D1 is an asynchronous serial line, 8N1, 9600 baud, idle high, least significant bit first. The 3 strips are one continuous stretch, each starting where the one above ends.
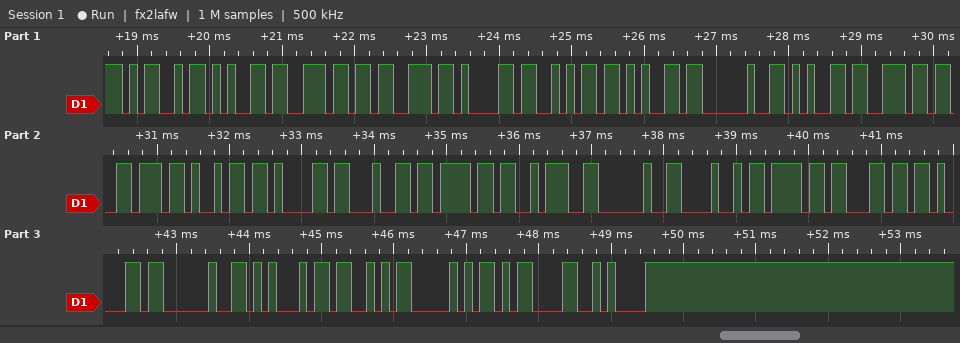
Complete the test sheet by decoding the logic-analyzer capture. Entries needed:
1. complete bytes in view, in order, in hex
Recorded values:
4D 65 6E 73 61 6A 65 20 65 6E 76 69 61 64 6F 3A 20 48 6F 6C 61 20 45 53 50 0D 0A
